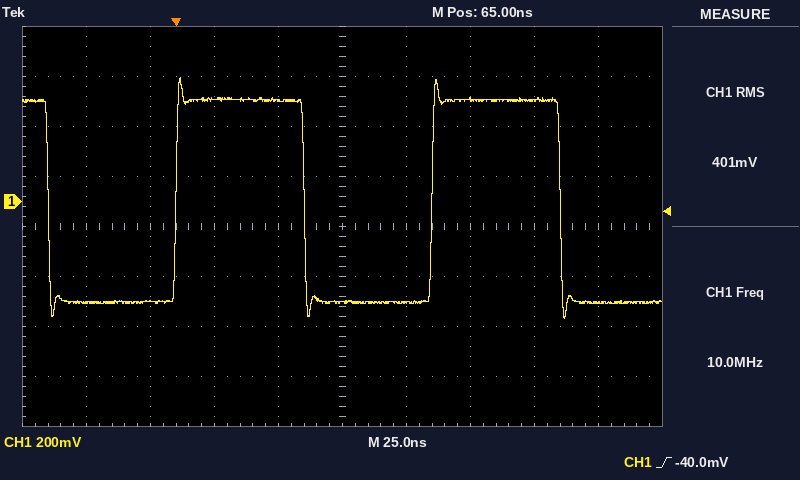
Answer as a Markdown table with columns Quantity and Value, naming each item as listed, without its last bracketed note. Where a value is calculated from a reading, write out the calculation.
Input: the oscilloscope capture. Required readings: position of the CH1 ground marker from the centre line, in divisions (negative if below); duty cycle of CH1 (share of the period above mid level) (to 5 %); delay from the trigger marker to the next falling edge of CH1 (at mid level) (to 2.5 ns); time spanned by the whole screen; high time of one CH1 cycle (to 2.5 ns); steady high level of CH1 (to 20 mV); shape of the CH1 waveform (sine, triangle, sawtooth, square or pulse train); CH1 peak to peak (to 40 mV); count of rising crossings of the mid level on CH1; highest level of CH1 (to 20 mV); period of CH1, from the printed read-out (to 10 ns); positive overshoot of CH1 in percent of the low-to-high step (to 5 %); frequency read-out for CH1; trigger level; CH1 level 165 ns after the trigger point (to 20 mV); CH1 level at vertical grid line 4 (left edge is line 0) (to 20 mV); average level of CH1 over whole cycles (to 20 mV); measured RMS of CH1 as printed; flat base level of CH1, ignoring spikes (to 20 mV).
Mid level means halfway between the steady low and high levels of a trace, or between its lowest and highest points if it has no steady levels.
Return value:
| Quantity | Value |
|---|---|
| position of the CH1 ground marker from the centre line, in divisions | +0.5 div |
| duty cycle of CH1 (share of the period above mid level) | 50 % |
| delay from the trigger marker to the next falling edge of CH1 (at mid level) | 50.0 ns |
| time spanned by the whole screen | 250 ns |
| high time of one CH1 cycle | 50.0 ns |
| steady high level of CH1 | 400 mV |
| shape of the CH1 waveform | square |
| CH1 peak to peak | 960 mV |
| count of rising crossings of the mid level on CH1 | 2 |
| highest level of CH1 | 500 mV |
| period of CH1, from the printed read-out | 1 / 10.0 MHz ≈ 100 ns |
| positive overshoot of CH1 in percent of the low-to-high step | 10 % |
| frequency read-out for CH1 | 10.0 MHz |
| trigger level | -40.0 mV |
| CH1 level 165 ns after the trigger point | -400 mV |
| CH1 level at vertical grid line 4 (left edge is line 0) | 400 mV |
| average level of CH1 over whole cycles | -400 mV + 0.5 × (400 mV − (-400 mV)) ≈ 0 mV |
| measured RMS of CH1 as printed | 401 mV |
| flat base level of CH1, ignoring spikes | -400 mV |
